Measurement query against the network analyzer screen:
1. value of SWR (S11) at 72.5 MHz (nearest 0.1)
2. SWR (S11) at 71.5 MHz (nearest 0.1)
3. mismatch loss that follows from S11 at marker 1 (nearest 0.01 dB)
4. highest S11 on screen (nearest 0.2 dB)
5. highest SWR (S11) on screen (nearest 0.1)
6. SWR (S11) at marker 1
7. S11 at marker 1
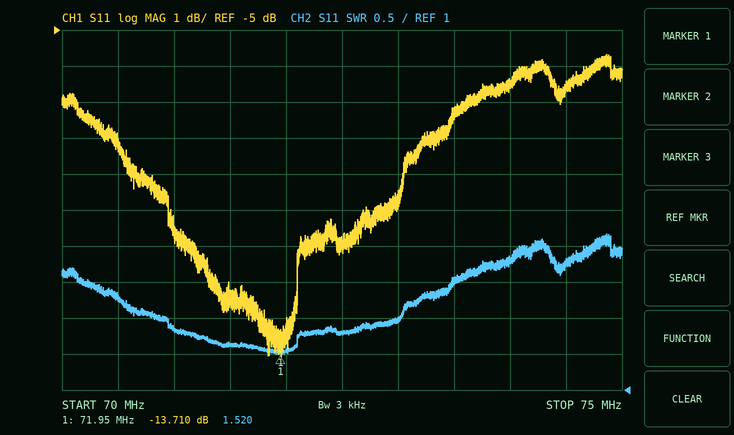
1.8
1.6
0.19 dB
-5.6 dB
3.2
1.520
-13.710 dB
